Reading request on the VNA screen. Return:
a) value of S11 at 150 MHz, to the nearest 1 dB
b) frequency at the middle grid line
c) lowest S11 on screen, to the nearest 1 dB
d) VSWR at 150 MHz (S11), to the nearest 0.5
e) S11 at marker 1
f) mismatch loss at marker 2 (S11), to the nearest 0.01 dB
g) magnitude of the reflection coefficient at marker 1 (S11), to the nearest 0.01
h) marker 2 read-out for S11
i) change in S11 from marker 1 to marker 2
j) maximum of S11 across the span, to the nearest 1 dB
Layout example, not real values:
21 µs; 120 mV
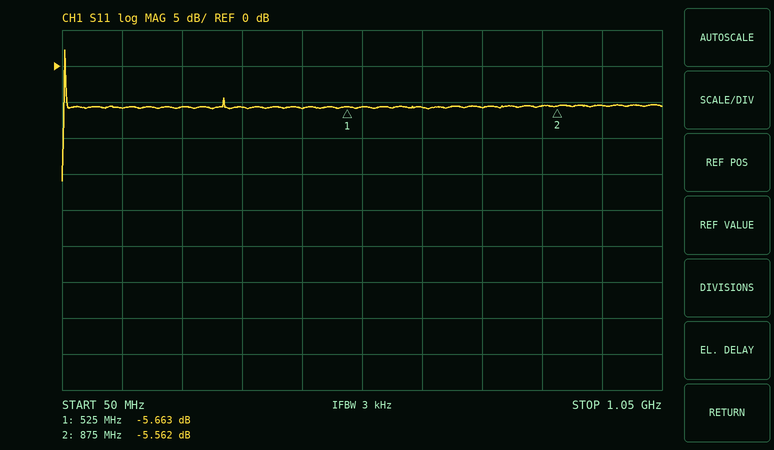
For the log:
-6 dB; 550 MHz; -16 dB; 3.0; -5.663 dB; 1.41 dB; 0.52; -5.562 dB; 0.101 dB; 2 dB
